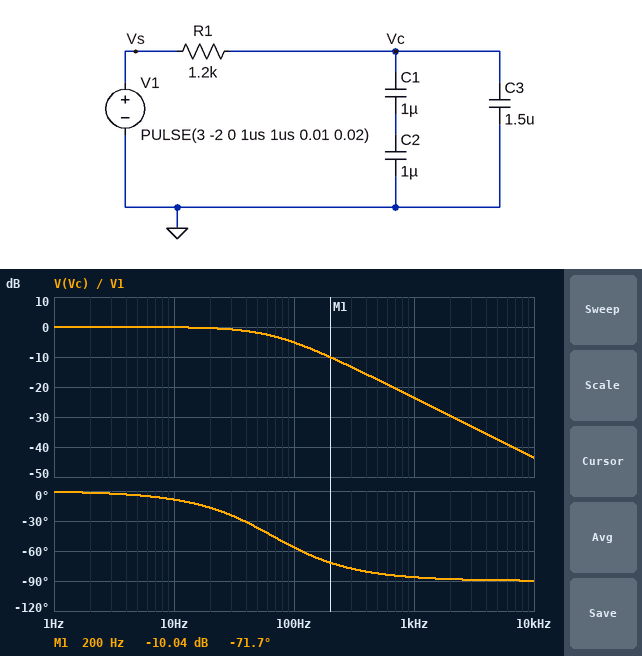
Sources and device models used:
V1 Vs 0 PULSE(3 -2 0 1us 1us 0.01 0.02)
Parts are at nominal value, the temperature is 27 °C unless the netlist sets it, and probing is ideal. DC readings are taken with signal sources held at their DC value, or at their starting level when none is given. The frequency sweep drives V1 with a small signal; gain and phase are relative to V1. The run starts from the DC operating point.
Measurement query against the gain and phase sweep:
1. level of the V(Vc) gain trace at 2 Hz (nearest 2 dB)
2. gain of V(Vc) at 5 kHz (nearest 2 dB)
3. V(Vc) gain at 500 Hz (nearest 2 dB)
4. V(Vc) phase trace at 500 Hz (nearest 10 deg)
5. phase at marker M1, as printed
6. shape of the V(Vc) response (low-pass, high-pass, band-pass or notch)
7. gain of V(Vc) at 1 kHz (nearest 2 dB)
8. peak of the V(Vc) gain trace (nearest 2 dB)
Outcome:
0 dB
-38 dB
-18 dB
-80 deg
-71.7 deg
low-pass
-24 dB
0 dB
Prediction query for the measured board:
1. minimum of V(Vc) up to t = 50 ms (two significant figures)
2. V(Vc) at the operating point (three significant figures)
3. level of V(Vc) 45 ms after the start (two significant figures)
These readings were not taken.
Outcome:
-1.9 V
3.00 V
-1.4 V
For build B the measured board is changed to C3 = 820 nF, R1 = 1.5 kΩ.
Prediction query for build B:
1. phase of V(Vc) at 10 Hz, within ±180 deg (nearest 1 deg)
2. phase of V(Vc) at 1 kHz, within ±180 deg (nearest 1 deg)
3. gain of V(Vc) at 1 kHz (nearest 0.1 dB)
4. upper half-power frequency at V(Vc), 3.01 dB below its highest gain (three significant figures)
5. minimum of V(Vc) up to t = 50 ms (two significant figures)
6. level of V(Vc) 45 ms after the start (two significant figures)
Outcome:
-7 deg
-85 deg
-21.9 dB
80.4 Hz
-2.0 V
-1.6 V
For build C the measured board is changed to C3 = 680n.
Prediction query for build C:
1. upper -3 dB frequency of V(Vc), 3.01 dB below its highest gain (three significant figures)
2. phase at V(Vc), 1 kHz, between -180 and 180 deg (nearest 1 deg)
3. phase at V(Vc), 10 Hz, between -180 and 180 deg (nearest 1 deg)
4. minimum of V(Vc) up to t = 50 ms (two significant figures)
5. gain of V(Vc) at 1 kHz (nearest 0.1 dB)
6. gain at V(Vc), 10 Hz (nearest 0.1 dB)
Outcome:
112 Hz
-84 deg
-5 deg
-2.0 V
-19.0 dB
0 dB
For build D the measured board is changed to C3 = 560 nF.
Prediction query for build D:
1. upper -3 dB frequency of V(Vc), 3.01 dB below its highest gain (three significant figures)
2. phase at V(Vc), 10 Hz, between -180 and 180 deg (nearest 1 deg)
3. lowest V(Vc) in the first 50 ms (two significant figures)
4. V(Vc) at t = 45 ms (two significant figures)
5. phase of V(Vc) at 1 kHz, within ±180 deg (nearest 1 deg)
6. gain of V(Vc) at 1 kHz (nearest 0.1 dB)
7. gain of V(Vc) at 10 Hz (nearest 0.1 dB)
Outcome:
125 Hz
-5 deg
-2.0 V
-1.9 V
-83 deg
-18.1 dB
0 dB
